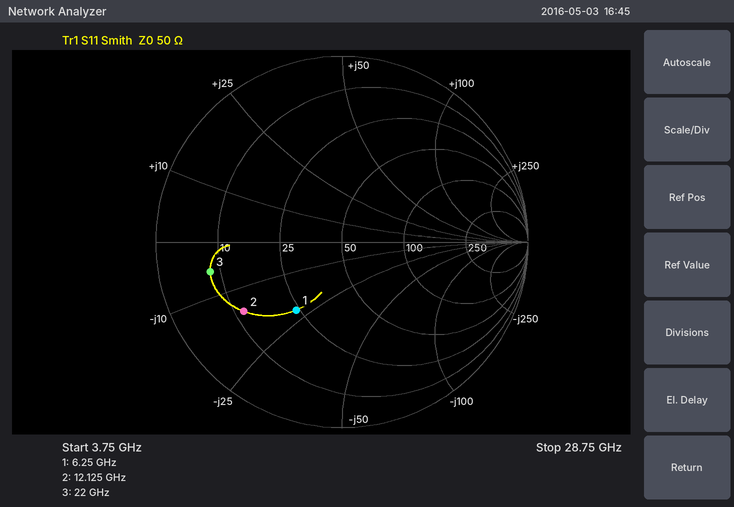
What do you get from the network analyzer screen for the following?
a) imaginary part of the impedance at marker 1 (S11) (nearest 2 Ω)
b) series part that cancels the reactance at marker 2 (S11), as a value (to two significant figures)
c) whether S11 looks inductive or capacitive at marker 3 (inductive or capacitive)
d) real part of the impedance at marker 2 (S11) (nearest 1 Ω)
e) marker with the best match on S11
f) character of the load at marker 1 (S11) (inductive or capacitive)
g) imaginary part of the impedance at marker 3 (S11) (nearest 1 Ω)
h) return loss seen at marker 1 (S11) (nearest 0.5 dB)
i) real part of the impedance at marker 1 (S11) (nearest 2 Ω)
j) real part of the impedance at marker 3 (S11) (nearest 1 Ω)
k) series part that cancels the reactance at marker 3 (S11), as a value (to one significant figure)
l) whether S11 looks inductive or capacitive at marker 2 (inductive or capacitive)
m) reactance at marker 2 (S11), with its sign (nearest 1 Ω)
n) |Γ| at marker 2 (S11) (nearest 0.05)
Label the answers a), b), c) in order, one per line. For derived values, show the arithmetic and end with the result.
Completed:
a) -22 Ω
b) L = 15 Ω/(2π × 12.125 GHz) ≈ 197 pH, so 200 pH to two significant figures
c) capacitive
d) 12 Ω
e) marker 1
f) capacitive
g) -5 Ω
h) 7.0 dB
i) 24 Ω
j) 8 Ω
k) L = 5 Ω/(2π × 22 GHz) ≈ 36.2 pH, so 40 pH to one significant figure
l) capacitive
m) -15 Ω
n) 0.65
